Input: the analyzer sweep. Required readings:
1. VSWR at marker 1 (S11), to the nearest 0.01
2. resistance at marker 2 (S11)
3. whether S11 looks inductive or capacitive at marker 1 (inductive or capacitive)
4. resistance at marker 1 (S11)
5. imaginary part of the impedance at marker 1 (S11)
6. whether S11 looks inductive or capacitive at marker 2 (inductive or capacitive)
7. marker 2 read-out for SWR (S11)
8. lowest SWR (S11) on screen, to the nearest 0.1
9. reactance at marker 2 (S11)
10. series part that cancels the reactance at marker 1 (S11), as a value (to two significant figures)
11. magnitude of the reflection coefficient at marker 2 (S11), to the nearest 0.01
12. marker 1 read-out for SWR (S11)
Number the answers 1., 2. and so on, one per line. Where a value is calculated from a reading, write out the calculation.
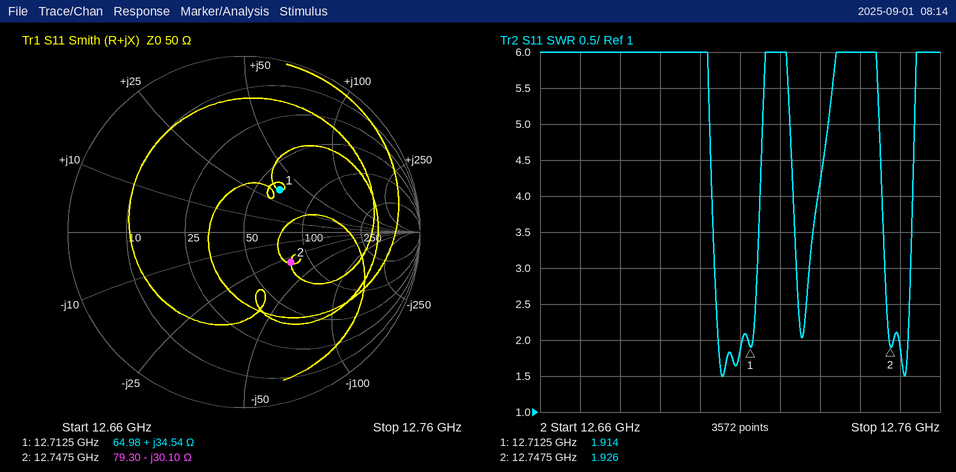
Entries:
1. 1.91
2. 79.30 Ω
3. inductive
4. 64.98 Ω
5. +34.54 Ω
6. capacitive
7. 1.926
8. 1.5
9. -30.10 Ω
10. C = 1/(2π × 12.7125 GHz × 34.54 Ω) ≈ 362 fF, so 360 fF to two significant figures
11. 0.32
12. 1.914
